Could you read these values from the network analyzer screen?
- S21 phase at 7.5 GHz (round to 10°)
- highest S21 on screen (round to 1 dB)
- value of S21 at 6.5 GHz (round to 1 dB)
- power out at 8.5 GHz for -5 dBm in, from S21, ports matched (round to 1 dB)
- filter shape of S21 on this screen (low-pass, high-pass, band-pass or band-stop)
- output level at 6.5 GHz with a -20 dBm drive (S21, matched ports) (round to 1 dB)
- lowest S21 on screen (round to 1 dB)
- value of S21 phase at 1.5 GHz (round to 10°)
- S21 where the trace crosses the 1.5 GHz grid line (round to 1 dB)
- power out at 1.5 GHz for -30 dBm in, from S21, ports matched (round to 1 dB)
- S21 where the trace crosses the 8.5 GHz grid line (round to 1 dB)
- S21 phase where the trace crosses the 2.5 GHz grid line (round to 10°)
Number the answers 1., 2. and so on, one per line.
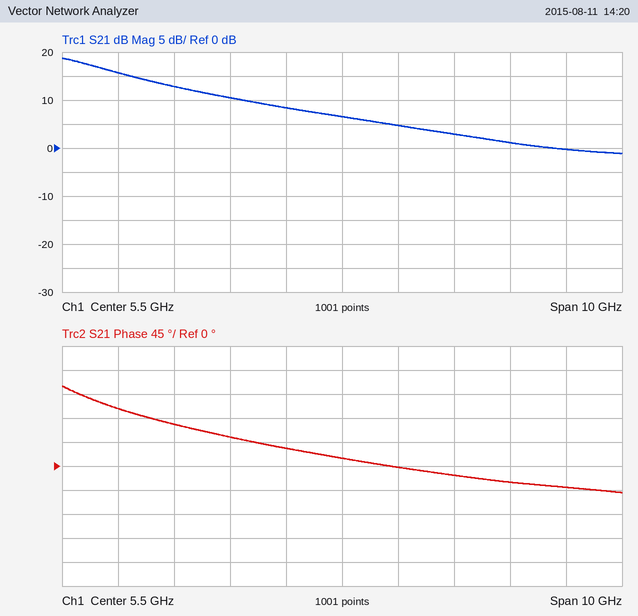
1. -20°
2. 19 dB
3. 5 dB
4. -4 dBm
5. low-pass
6. -15 dBm
7. -1 dB
8. 110°
9. 16 dB
10. -14 dBm
11. 1 dB
12. 80°
